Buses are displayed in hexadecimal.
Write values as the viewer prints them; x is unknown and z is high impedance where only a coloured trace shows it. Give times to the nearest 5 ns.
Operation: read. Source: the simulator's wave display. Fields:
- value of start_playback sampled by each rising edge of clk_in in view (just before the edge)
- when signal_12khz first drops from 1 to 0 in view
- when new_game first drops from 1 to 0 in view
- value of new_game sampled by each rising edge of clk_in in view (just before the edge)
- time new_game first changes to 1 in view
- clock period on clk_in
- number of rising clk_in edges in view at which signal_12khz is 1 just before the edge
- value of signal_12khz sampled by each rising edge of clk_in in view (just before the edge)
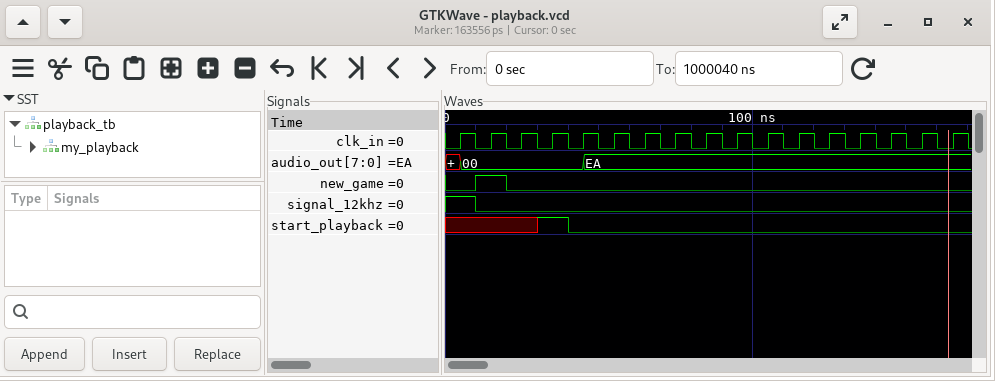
x x x 1 0 0 0 0 0 0 0 0 0 0 0 0 0
10 ns
20 ns
0 1 0 0 0 0 0 0 0 0 0 0 0 0 0 0 0
10 ns
10 ns
1
1 0 0 0 0 0 0 0 0 0 0 0 0 0 0 0 0
